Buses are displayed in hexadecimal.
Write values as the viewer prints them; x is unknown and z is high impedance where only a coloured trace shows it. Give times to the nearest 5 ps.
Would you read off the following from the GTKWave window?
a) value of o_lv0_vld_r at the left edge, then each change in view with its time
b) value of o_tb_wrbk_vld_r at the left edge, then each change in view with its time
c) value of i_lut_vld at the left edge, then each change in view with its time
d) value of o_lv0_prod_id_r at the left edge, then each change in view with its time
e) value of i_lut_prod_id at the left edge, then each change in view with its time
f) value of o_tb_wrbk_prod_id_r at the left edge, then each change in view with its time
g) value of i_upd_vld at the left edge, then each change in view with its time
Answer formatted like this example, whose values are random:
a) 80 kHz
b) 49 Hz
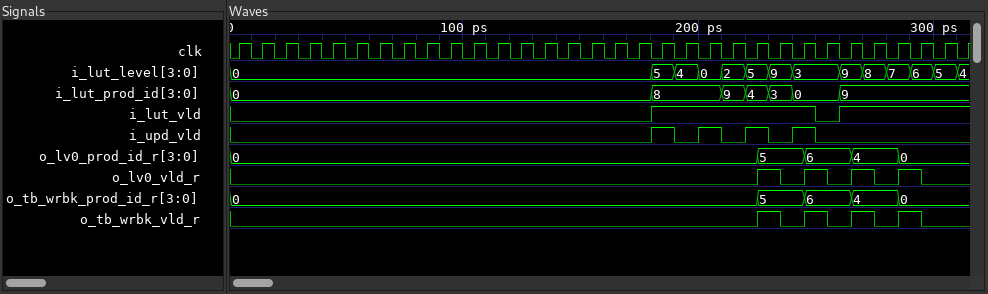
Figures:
a) 0, 1 at 225 ps, 0 at 235 ps, 1 at 245 ps, 0 at 255 ps, 1 at 265 ps, 0 at 275 ps, 1 at 285 ps, 0 at 295 ps
b) 0, 1 at 225 ps, 0 at 235 ps, 1 at 245 ps, 0 at 255 ps, 1 at 265 ps, 0 at 275 ps, 1 at 285 ps, 0 at 295 ps
c) 0, 1 at 180 ps, 0 at 250 ps, 1 at 260 ps
d) 0, 5 at 225 ps, 6 at 245 ps, 4 at 265 ps, 0 at 285 ps
e) 0, 8 at 180 ps, 9 at 210 ps, 4 at 220 ps, 3 at 230 ps, 0 at 240 ps, 9 at 260 ps
f) 0, 5 at 225 ps, 6 at 245 ps, 4 at 265 ps, 0 at 285 ps
g) 0, 1 at 180 ps, 0 at 190 ps, 1 at 200 ps, 0 at 210 ps, 1 at 220 ps, 0 at 230 ps, 1 at 240 ps, 0 at 250 ps
